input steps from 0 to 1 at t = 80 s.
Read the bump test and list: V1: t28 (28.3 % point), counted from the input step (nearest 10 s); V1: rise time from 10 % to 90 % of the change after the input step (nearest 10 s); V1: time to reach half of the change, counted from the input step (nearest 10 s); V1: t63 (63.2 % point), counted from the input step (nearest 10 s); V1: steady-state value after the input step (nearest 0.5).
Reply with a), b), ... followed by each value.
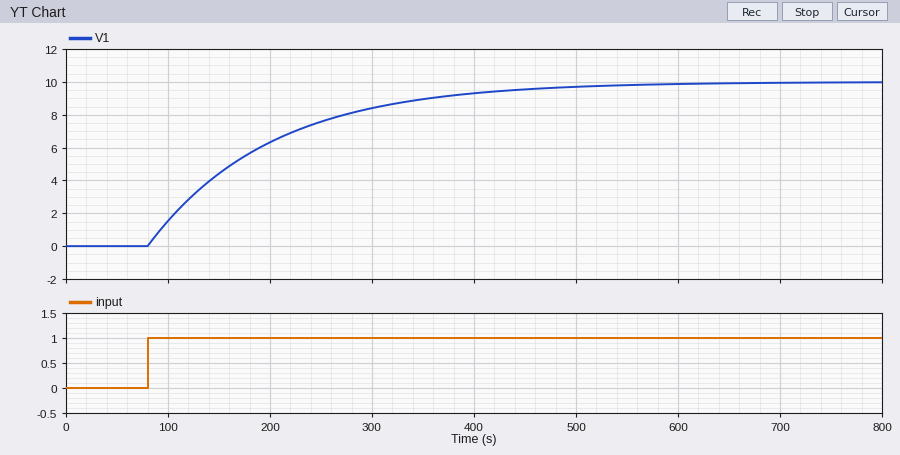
a) 40 s
b) 260 s
c) 80 s
d) 120 s
e) 10.0
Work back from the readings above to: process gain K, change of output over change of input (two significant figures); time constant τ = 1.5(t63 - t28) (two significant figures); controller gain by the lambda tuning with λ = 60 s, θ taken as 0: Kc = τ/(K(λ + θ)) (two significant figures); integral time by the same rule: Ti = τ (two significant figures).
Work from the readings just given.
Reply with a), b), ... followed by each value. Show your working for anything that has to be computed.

a) (10 - 0) / 1 = 10
b) 1.5 × (120 - 40) = 120 s
c) 120 / (10 × (60 + 0)) = 0.20
d) 120 s
